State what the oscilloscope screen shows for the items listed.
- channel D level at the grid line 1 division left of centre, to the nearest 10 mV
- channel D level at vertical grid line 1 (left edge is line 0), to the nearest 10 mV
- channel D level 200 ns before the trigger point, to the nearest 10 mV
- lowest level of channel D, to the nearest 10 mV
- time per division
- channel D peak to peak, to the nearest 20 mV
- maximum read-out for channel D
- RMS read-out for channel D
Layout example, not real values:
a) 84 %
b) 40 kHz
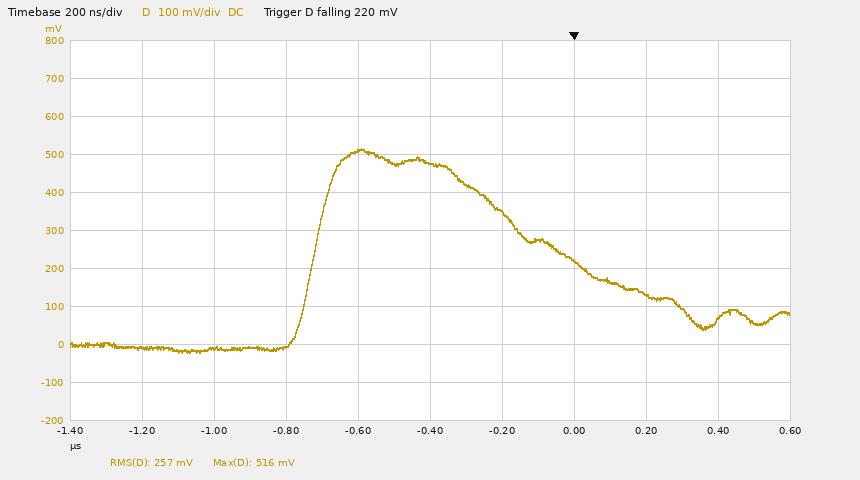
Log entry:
a) 510 mV
b) -10 mV
c) 350 mV
d) -20 mV
e) 200 ns
f) 540 mV
g) 516 mV
h) 257 mV
